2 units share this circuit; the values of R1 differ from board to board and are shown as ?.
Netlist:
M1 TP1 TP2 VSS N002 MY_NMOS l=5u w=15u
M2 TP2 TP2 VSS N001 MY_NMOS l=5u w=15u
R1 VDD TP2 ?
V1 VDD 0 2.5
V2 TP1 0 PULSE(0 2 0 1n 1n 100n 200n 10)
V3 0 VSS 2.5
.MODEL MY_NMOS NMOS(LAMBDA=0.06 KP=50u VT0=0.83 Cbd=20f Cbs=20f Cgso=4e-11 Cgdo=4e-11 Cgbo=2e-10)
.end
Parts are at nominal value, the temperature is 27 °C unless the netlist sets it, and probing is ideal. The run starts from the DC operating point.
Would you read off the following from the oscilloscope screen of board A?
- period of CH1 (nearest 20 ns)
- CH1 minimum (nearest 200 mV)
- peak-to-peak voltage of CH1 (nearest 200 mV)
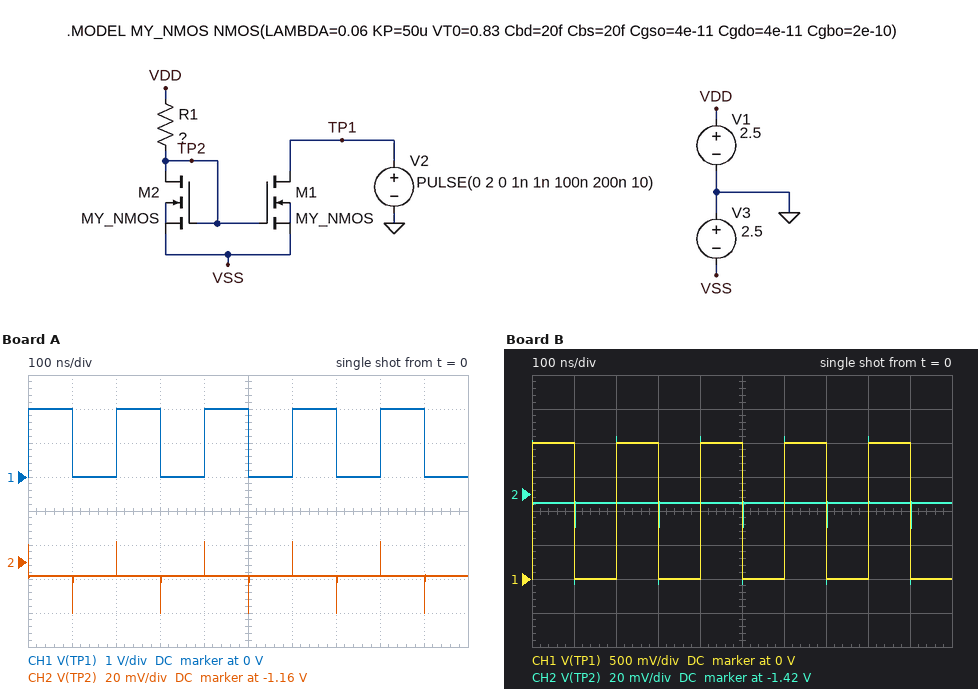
200 ns
0 V
2.0 V
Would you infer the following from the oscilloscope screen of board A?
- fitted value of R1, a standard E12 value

180 kΩ
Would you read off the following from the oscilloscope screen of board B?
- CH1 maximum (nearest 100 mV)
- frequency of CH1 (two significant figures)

2.0 V
5.0 MHz
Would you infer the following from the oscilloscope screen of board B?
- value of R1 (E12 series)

820 kΩ
